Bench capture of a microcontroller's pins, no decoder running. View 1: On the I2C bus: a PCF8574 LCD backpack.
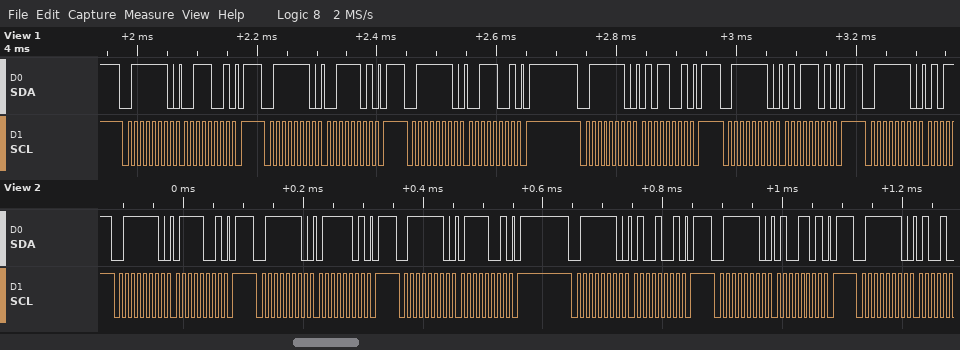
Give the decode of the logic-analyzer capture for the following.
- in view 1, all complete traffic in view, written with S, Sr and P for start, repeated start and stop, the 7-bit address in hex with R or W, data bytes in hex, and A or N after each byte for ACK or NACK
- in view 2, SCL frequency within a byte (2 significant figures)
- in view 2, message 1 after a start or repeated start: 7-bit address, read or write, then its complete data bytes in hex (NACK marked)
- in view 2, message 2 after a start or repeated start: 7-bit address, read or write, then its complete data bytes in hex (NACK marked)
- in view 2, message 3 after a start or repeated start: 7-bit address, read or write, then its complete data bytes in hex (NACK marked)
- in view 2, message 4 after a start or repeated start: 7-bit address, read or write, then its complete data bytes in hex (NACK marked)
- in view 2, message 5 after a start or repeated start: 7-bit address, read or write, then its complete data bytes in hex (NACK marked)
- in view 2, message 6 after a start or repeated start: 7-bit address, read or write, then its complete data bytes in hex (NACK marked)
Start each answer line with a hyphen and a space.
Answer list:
- S 3FW A 39 A P S 3FW A 3D A P S 3FW A 39 A P S 3FW A 59 A P S 3FW A 5D A P S 3FW A
- 100 kHz
- 0x3F write: 79
- 0x3F write: 7D
- 0x3F write: 79
- 0x3F write: 49
- 0x3F write: 4D
- 0x3F write
